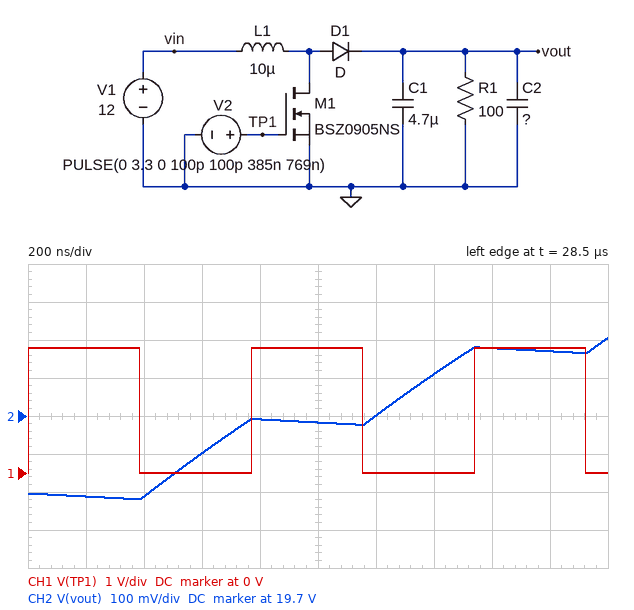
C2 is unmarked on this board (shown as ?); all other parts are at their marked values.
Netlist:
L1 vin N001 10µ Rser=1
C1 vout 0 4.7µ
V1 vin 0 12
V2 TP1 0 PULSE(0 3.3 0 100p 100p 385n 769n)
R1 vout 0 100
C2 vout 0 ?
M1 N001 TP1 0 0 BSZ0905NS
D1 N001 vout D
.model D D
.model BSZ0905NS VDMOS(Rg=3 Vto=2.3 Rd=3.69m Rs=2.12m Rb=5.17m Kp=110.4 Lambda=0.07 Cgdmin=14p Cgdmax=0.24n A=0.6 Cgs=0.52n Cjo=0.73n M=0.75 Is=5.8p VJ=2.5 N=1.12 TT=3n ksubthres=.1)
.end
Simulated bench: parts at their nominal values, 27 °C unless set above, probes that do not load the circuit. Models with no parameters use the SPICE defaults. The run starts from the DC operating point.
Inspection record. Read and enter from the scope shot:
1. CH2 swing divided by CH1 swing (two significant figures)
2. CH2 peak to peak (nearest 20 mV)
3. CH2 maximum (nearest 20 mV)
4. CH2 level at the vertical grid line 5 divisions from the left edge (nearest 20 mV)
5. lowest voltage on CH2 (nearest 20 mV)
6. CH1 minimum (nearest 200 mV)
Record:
0.13
420 mV
19.90 V
19.68 V
19.48 V
0 V
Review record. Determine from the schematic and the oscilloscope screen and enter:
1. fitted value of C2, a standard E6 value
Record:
150 nF
